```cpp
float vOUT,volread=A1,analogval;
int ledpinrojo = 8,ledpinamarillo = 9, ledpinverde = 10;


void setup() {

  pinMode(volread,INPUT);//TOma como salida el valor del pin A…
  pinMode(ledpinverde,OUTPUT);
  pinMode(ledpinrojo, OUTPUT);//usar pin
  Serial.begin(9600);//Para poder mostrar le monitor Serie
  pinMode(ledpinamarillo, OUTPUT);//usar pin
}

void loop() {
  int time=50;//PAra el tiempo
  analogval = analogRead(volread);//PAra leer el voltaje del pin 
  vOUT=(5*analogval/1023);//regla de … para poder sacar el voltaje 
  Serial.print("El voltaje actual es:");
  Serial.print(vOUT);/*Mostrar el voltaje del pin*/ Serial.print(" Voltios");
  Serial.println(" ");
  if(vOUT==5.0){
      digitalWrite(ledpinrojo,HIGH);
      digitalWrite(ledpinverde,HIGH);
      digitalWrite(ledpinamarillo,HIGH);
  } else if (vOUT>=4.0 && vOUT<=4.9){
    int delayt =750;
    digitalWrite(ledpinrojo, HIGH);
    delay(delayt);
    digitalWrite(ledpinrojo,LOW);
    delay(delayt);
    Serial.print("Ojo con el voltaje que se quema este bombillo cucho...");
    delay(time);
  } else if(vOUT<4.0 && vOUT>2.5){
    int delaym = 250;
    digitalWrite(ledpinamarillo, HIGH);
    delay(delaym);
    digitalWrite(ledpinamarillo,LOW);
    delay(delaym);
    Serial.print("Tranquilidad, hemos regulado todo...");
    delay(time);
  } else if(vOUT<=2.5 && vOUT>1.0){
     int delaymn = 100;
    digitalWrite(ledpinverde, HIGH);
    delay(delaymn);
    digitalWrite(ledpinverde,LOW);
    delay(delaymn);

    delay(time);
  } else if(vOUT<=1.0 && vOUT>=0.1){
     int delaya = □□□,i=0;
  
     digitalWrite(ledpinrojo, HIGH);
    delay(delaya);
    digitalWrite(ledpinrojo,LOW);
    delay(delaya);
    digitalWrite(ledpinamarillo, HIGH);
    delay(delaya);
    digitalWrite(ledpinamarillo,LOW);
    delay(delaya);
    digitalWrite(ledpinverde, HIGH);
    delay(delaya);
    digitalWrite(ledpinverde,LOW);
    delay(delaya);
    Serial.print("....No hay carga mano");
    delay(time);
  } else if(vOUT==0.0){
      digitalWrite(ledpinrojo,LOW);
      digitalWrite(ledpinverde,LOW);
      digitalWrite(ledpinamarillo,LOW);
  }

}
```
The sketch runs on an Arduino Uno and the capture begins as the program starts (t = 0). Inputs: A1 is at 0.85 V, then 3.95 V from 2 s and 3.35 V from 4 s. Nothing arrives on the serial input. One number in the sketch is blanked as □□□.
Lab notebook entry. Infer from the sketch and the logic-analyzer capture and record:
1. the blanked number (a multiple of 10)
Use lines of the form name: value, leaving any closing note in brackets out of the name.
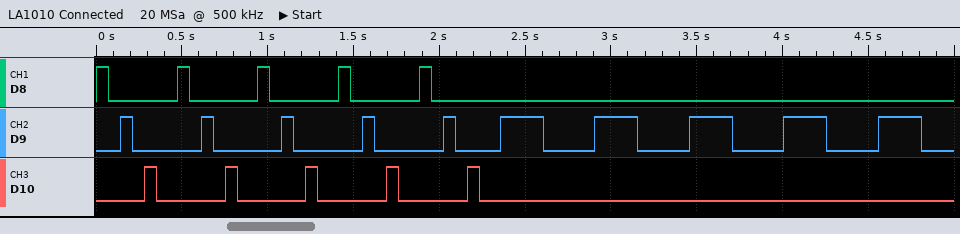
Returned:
the blanked number: 70
